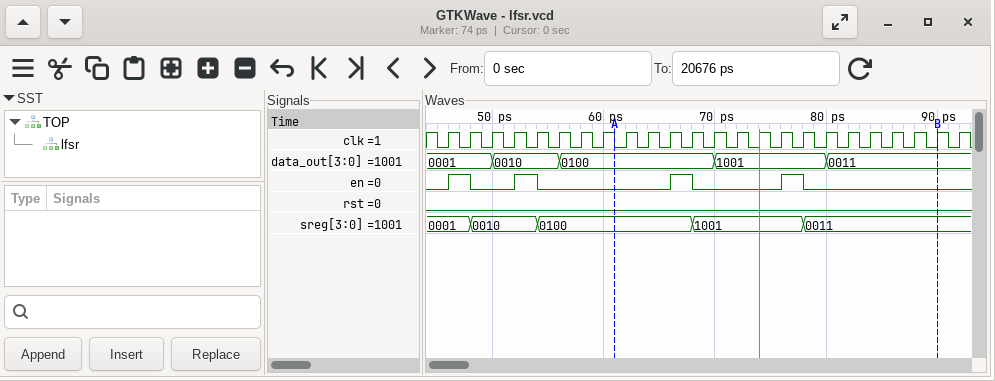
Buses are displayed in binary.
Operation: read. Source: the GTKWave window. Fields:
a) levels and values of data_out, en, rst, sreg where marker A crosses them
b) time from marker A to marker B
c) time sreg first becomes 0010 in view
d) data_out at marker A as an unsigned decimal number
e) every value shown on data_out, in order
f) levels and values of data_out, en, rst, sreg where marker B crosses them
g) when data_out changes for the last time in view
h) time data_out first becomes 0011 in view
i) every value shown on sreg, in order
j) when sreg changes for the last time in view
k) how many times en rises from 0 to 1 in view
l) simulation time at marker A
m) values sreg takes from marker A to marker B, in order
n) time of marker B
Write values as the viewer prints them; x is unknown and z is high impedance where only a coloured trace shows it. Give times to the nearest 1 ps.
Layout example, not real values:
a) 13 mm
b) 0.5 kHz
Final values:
a) data_out=0100, en=0, rst=0, sreg=0100
b) 29 ps
c) 48 ps
d) 4
e) 0001, 0010, 0100, 1001, 0011
f) data_out=0011, en=0, rst=0, sreg=0011
g) 80 ps
h) 80 ps
i) 0001, 0010, 0100, 1001, 0011
j) 78 ps
k) 4
l) 61 ps
m) 0100, 1001, 0011
n) 90 ps
